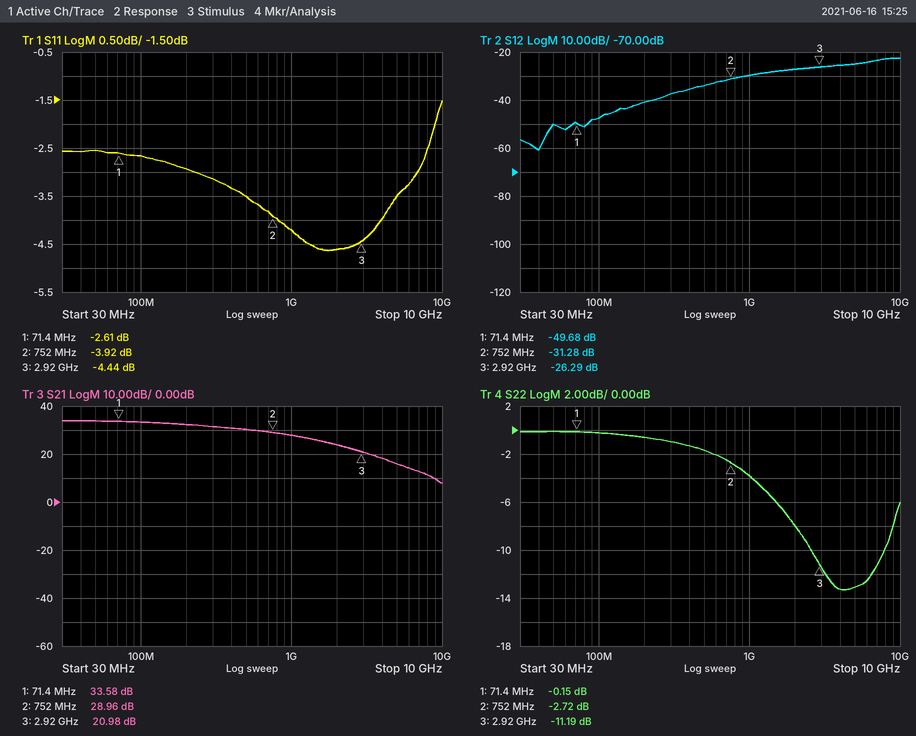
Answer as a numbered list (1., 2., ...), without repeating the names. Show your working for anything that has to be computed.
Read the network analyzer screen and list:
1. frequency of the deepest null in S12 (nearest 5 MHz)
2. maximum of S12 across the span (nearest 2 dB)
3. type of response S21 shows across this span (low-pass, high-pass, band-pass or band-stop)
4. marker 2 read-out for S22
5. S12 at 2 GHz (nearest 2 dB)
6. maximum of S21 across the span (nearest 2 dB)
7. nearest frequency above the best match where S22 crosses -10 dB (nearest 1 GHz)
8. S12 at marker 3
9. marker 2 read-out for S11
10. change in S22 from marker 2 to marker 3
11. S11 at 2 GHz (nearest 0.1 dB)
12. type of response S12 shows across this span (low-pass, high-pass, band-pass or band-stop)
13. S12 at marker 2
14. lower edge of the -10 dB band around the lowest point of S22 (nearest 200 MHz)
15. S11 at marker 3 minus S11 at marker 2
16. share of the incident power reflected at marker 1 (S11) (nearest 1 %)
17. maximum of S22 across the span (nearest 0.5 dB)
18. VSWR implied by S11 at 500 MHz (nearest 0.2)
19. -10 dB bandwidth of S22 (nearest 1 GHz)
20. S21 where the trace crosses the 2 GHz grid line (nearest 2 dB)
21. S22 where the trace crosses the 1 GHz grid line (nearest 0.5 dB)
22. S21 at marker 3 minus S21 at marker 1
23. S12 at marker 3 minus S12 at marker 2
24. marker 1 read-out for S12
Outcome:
1. 40 MHz
2. -22 dB
3. low-pass
4. -2.72 dB
5. -28 dB
6. 34 dB
7. 8 GHz
8. -26.29 dB
9. -3.92 dB
10. -11.19 − (-2.72) = -8.47 dB
11. -4.6 dB
12. high-pass
13. -31.28 dB
14. 2.6 GHz
15. -4.44 − (-3.92) = -0.52 dB
16. 10^(-2.61/10) ≈ 55 %
17. 0.0 dB
18. |Γ| = 10^(-3.5/20) = 0.6683; VSWR = (1 + 0.6683)/(1 − 0.6683) ≈ 5.0
19. 8 GHz − 2.6 GHz = 5.4 GHz
20. 24 dB
21. -4.0 dB
22. 20.98 − (33.58) = -12.60 dB
23. -26.29 − (-31.28) = 4.99 dB
24. -49.68 dB
